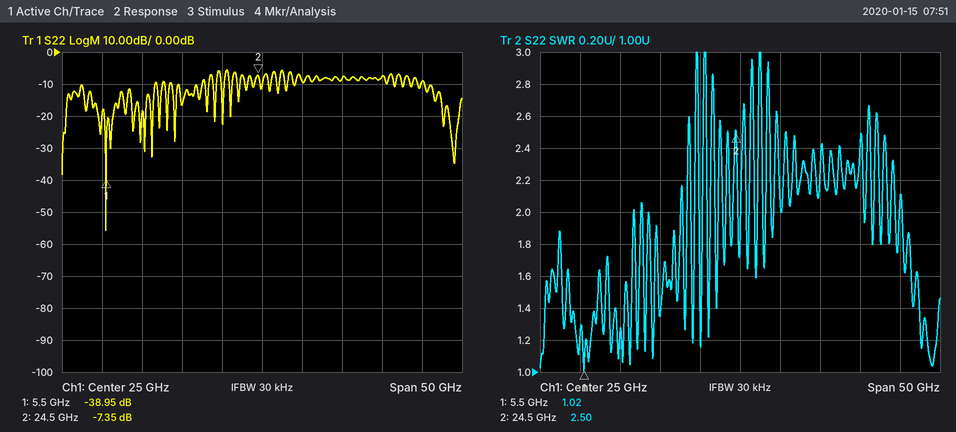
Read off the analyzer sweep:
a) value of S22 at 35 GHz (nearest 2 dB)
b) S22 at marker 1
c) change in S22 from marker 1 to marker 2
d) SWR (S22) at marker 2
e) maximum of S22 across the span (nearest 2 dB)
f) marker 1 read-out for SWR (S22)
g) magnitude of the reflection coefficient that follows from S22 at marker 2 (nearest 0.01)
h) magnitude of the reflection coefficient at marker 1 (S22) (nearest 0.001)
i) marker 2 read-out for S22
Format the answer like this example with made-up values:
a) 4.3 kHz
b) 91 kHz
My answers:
a) -8 dB
b) -38.95 dB
c) 31.60 dB
d) 2.50
e) -6 dB
f) 1.02
g) 0.43
h) 0.011
i) -7.35 dB
